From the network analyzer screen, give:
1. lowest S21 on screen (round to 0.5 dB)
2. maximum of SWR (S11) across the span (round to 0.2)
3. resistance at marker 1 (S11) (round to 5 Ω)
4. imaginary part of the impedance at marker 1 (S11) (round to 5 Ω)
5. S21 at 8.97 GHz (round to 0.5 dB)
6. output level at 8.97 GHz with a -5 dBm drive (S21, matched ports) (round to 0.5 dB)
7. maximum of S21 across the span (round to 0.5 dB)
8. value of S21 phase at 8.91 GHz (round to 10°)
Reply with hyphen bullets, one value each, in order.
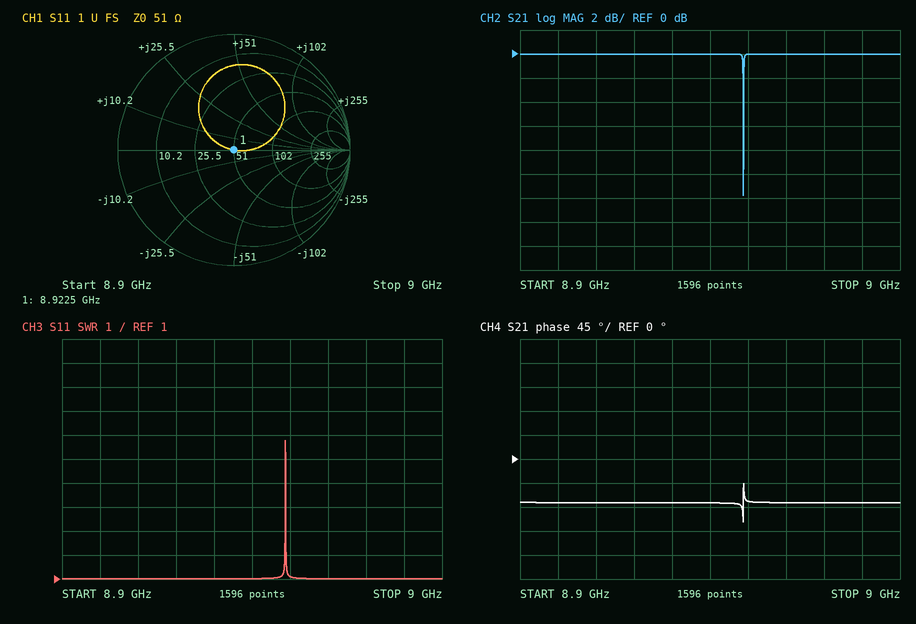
- -12.0 dB
- 6.8
- 50 Ω
- 0 Ω
- 0.0 dB
- -5.0 dBm
- 0.0 dB
- -80°
